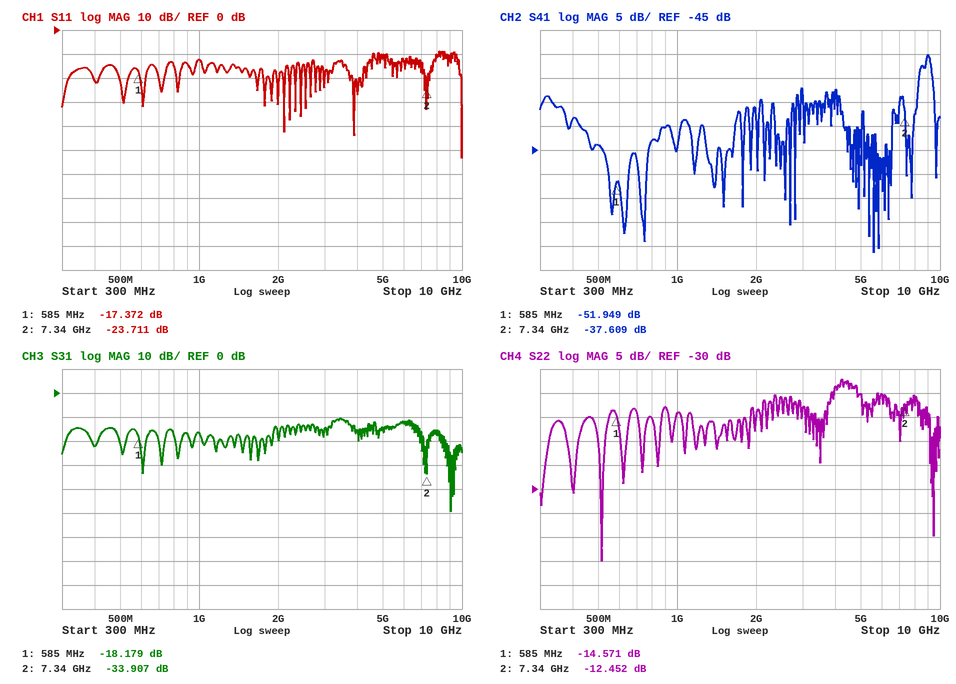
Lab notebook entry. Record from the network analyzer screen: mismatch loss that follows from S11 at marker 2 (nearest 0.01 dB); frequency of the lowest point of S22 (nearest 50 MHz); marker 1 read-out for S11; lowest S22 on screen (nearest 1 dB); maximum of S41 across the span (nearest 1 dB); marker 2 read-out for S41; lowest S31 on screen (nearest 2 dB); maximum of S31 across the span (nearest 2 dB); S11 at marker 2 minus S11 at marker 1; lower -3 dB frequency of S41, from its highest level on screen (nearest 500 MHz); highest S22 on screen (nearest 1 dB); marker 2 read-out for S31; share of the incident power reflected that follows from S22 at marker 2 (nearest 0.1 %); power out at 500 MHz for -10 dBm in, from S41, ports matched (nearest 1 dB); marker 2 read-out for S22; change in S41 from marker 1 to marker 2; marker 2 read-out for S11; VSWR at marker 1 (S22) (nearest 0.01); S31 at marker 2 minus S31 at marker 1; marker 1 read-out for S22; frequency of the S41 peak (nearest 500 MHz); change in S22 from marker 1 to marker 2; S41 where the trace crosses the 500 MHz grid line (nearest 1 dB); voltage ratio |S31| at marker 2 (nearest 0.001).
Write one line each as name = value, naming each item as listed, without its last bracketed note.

mismatch loss that follows from S11 at marker 2 = 0.02 dB
frequency of the lowest point of S22 = 500 MHz
marker 1 read-out for S11 = -17.372 dB
lowest S22 on screen = -45 dB
maximum of S41 across the span = -25 dB
marker 2 read-out for S41 = -37.609 dB
lowest S31 on screen = -50 dB
maximum of S31 across the span = -10 dB
S11 at marker 2 minus S11 at marker 1 = -6.339 dB
lower -3 dB frequency of S41, from its highest level on screen = 8.5 GHz
highest S22 on screen = -7 dB
marker 2 read-out for S31 = -33.907 dB
share of the incident power reflected that follows from S22 at marker 2 = 5.7 %
power out at 500 MHz for -10 dBm in, from S41, ports matched = -54 dBm
marker 2 read-out for S22 = -12.452 dB
change in S41 from marker 1 to marker 2 = 14.340 dB
marker 2 read-out for S11 = -23.711 dB
VSWR at marker 1 (S22) = 1.46
S31 at marker 2 minus S31 at marker 1 = -15.728 dB
marker 1 read-out for S22 = -14.571 dB
frequency of the S41 peak = 9.0 GHz
change in S22 from marker 1 to marker 2 = 2.119 dB
S41 where the trace crosses the 500 MHz grid line = -44 dB
voltage ratio |S31| at marker 2 = 0.020
